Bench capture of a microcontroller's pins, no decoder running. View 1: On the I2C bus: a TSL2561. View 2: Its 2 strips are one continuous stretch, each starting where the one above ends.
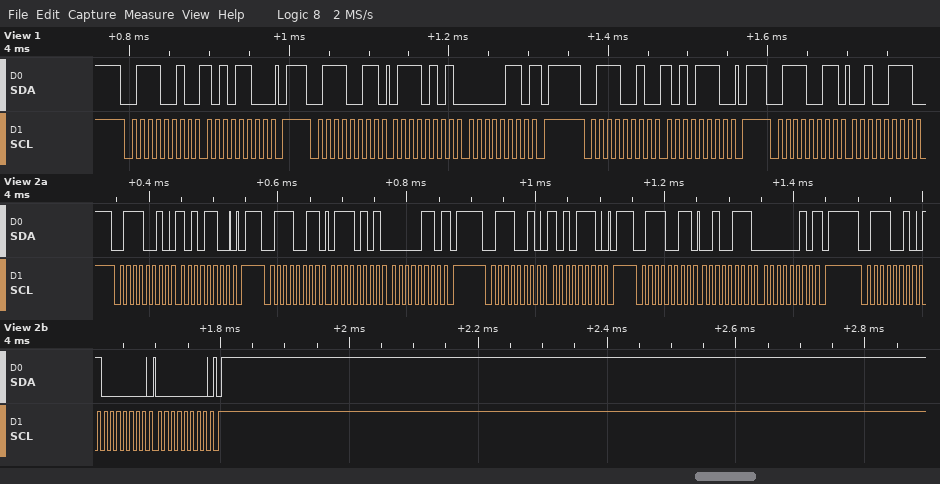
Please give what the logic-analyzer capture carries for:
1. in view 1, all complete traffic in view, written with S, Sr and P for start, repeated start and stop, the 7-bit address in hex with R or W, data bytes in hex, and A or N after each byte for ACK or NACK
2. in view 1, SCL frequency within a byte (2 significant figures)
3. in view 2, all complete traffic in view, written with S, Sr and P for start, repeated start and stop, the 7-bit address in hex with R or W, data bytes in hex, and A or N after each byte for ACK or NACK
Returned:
S 39W A AC A P S 39R A 75 A 06 N P S 39W A AE A P S 39R A 27 A
100 kHz
S 39W A AC A P S 39R A 75 A 06 N P S 39W A AE A P S 39R A 27 A 02 N P S 39W A 80 A 00 A P
